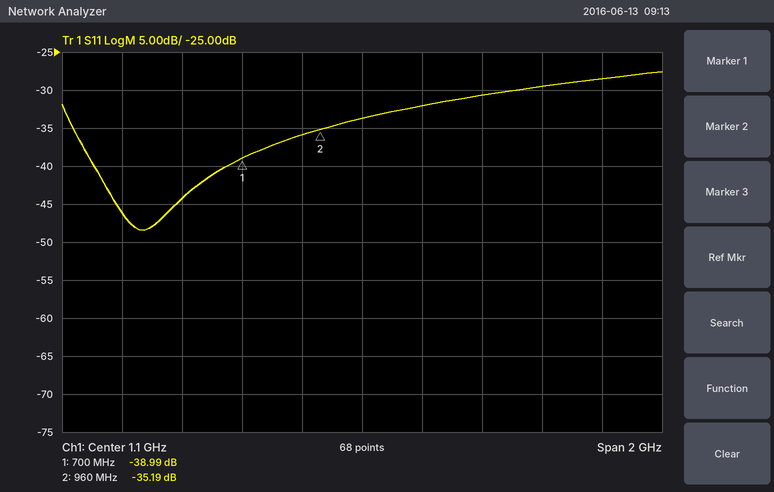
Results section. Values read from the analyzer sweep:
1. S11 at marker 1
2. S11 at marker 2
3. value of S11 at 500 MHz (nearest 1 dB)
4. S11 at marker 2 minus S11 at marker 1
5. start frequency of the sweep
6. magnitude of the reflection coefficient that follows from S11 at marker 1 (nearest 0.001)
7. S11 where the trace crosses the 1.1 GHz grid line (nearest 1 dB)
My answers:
-38.99 dB
-35.19 dB
-44 dB
3.80 dB
100 MHz
0.011
-34 dB
